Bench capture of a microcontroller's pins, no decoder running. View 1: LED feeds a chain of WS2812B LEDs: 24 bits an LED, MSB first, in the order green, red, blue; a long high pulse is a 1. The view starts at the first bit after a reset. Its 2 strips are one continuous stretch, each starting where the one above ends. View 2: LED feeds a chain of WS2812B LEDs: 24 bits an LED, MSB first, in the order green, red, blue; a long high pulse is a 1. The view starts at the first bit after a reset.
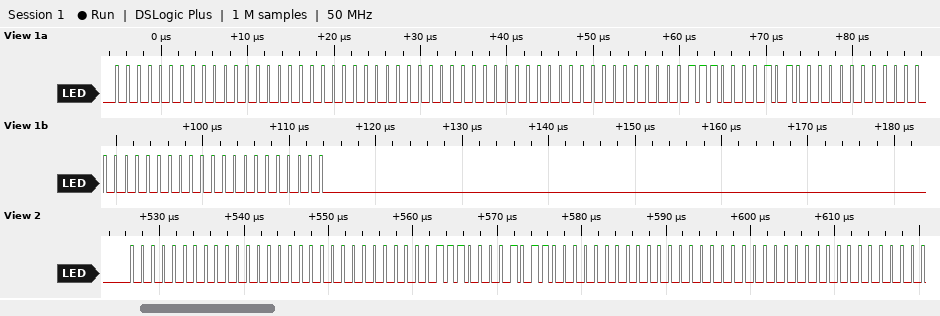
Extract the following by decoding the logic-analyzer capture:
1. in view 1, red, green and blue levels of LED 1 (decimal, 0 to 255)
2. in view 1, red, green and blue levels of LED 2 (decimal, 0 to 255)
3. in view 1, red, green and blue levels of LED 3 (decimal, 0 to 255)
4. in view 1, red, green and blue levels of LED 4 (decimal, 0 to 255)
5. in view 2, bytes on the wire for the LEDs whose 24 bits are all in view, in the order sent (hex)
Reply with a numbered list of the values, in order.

1. 0, 0, 0
2. 0, 0, 0
3. 10, 7, 0
4. 0, 0, 0
5. 00 00 00 07 0B 00 00 00 00
